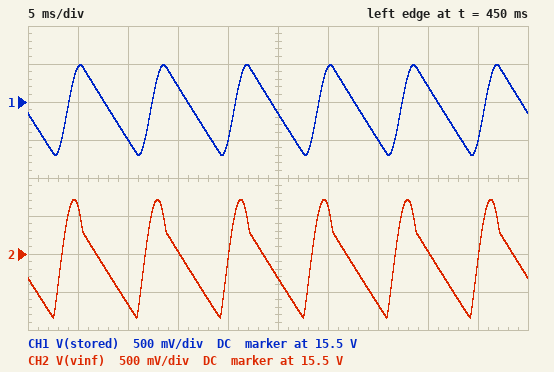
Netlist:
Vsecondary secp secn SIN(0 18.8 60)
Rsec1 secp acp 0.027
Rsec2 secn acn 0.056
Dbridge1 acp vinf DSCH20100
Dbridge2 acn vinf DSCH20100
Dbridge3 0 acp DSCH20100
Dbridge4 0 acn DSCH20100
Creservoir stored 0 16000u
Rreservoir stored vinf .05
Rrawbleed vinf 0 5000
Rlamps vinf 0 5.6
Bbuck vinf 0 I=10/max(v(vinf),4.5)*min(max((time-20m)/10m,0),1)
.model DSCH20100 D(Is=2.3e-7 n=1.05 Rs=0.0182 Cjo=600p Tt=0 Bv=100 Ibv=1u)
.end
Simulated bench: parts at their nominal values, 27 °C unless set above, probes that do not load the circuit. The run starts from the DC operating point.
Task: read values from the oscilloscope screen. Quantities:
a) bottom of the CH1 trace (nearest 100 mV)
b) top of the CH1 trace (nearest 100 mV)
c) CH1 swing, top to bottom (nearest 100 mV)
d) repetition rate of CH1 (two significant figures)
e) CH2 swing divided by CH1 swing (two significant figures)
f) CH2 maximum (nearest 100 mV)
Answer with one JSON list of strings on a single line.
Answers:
["14.8 V", "16.0 V", "1.2 V", "120 Hz", "1.3", "16.2 V"]
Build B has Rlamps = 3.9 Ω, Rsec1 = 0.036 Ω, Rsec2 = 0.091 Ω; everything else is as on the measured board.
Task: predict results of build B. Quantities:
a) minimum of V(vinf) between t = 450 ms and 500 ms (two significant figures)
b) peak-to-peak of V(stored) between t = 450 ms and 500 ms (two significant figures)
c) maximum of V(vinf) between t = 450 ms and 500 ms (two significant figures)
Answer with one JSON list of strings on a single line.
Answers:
["14 V", "1.4 V", "15 V"]
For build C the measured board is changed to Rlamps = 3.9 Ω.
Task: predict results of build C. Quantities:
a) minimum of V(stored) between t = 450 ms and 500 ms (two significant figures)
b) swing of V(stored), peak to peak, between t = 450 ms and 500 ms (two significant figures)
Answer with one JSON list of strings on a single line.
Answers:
["14 V", "1.5 V"]
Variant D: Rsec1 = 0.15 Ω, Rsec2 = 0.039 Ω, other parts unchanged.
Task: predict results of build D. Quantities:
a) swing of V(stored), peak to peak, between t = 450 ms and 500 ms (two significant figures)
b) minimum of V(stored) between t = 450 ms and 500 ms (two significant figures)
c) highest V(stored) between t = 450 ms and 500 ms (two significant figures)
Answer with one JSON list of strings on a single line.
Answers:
["1.1 V", "14 V", "15 V"]
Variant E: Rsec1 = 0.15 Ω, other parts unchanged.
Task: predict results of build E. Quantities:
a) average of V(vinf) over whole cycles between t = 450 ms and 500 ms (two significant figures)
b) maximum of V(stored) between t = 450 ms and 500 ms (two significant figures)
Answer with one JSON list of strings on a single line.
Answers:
["14 V", "15 V"]
